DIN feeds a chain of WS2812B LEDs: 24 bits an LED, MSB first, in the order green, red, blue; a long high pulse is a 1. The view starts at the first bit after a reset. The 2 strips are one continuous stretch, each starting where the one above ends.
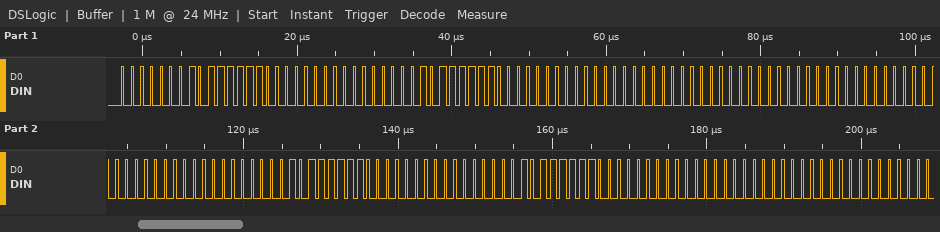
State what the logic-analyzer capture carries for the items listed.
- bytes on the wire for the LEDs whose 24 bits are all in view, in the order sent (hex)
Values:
01 7E 00 01 7E 00 00 00 00 00 00 00 01 7E 00 01 7E 00 00 00 00
